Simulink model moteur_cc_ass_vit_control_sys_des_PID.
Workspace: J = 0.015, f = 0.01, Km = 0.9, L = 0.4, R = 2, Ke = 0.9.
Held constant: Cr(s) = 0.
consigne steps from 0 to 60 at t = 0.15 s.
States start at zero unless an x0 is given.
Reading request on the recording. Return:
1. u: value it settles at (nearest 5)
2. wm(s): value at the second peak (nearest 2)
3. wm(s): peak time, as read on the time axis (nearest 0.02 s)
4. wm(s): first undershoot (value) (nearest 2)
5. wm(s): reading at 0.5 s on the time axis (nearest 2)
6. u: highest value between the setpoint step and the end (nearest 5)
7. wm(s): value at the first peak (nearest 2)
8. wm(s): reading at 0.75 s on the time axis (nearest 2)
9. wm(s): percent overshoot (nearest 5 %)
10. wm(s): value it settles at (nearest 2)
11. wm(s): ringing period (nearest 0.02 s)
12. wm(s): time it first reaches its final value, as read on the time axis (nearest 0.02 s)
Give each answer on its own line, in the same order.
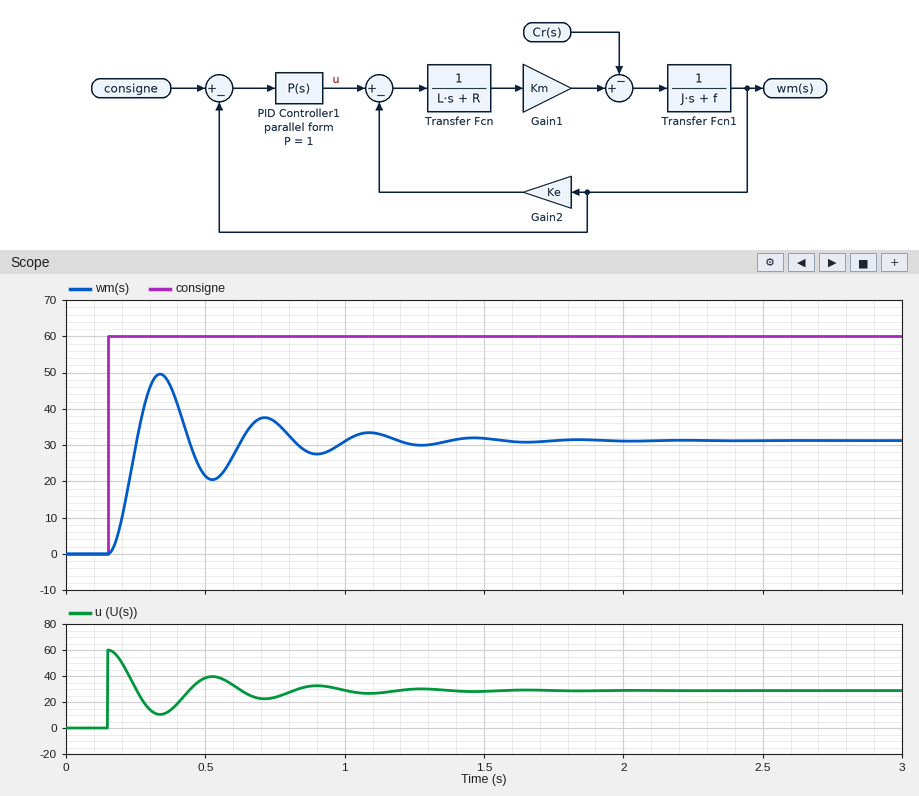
30
38
0.34 s
20
22
60
50
36
60 %
32
0.38 s
0.26 s
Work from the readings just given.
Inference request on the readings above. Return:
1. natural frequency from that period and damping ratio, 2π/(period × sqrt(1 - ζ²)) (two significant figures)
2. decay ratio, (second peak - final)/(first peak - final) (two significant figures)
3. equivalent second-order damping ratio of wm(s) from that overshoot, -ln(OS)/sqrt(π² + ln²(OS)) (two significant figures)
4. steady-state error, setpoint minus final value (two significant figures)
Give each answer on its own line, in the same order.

17 rad/s
0.33
0.16
28
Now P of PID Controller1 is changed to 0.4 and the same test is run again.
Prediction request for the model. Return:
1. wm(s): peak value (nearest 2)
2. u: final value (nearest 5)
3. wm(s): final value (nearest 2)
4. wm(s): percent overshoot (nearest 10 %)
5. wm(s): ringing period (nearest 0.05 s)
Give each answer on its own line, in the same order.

28
15
18
50 %
0.45 s
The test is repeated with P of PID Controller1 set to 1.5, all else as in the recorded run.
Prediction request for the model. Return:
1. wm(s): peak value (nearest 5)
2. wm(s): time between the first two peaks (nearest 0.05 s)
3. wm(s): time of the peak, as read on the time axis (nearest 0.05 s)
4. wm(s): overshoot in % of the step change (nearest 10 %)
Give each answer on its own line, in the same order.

60
0.35 s
0.30 s
60 %
